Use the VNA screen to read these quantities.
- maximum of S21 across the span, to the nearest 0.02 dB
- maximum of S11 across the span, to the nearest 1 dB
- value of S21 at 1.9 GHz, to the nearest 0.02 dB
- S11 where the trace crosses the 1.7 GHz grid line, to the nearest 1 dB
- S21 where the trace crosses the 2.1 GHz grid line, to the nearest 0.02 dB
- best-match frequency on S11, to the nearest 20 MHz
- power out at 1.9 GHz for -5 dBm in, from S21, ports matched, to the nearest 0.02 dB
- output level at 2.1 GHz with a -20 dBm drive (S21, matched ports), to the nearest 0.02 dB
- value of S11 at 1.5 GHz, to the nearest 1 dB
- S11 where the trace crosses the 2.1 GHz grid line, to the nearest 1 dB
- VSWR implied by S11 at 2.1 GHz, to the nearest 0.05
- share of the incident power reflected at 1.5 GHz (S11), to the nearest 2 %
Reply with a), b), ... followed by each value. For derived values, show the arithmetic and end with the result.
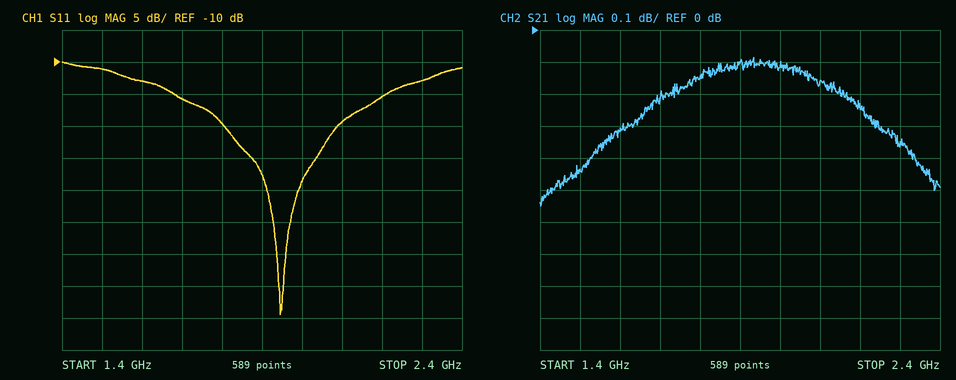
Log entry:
a) -0.08 dB
b) -10 dB
c) -0.10 dB
d) -16 dB
e) -0.16 dB
f) 1.94 GHz
g) -5 dBm + (-0.10 dB) = -5.10 dBm
h) -20 dBm + (-0.16 dB) = -20.16 dBm
i) -11 dB
j) -19 dB
k) |Γ| = 10^(-19/20) = 0.1122; VSWR = (1 + 0.1122)/(1 − 0.1122) ≈ 1.25
l) 10^(-11/10) ≈ 8 %
